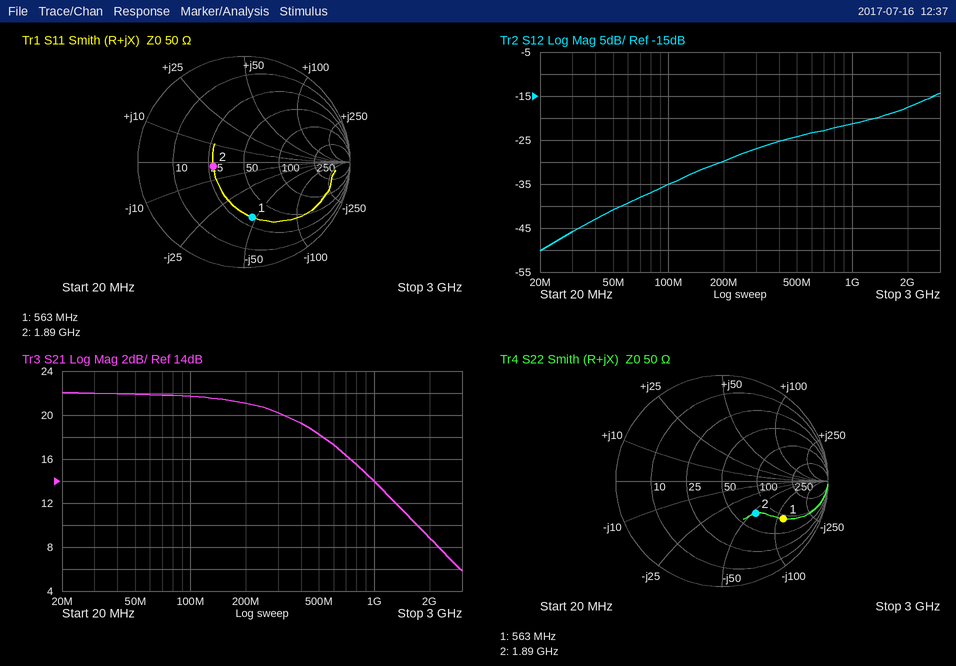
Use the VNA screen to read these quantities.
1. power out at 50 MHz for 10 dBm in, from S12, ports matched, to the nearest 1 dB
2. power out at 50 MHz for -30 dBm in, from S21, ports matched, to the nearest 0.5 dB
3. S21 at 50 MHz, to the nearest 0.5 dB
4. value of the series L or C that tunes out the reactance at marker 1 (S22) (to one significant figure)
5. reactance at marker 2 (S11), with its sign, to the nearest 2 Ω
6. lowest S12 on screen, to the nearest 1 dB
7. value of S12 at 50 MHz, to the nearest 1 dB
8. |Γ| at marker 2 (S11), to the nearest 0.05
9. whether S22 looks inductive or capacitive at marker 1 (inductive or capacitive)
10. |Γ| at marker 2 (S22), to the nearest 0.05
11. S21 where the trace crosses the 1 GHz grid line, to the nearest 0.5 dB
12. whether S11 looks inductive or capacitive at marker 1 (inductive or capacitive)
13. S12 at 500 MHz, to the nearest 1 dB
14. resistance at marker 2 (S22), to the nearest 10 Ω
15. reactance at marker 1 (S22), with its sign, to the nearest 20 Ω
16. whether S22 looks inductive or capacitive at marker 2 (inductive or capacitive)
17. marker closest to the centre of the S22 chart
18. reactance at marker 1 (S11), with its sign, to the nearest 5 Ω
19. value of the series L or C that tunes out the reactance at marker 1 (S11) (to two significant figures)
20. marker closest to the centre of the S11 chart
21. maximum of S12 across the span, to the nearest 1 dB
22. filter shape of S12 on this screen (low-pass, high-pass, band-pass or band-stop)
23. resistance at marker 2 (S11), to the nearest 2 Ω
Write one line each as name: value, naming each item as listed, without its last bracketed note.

power out at 50 MHz for 10 dBm in, from S12, ports matched, to the nearest 1 dB: -31 dBm
power out at 50 MHz for -30 dBm in, from S21, ports matched, to the nearest 0.5 dB: -8.0 dBm
S21 at 50 MHz, to the nearest 0.5 dB: 22.0 dB
value of the series L or C that tunes out the reactance at marker 1 (S22): 30 nH
reactance at marker 2 (S11), with its sign, to the nearest 2 Ω: -2 Ω
lowest S12 on screen, to the nearest 1 dB: -50 dB
value of S12 at 50 MHz, to the nearest 1 dB: -41 dB
|Γ| at marker 2 (S11), to the nearest 0.05: 0.30
whether S22 looks inductive or capacitive at marker 1: capacitive
|Γ| at marker 2 (S22), to the nearest 0.05: 0.45
S21 where the trace crosses the 1 GHz grid line, to the nearest 0.5 dB: 14.0 dB
whether S11 looks inductive or capacitive at marker 1: capacitive
S12 at 500 MHz, to the nearest 1 dB: -24 dB
resistance at marker 2 (S22), to the nearest 10 Ω: 70 Ω
reactance at marker 1 (S22), with its sign, to the nearest 20 Ω: -120 Ω
whether S22 looks inductive or capacitive at marker 2: capacitive
marker closest to the centre of the S22 chart: marker 2
reactance at marker 1 (S11), with its sign, to the nearest 5 Ω: -45 Ω
value of the series L or C that tunes out the reactance at marker 1 (S11): 13 nH
marker closest to the centre of the S11 chart: marker 2
maximum of S12 across the span, to the nearest 1 dB: -14 dB
filter shape of S12 on this screen: high-pass
resistance at marker 2 (S11), to the nearest 2 Ω: 28 Ω
